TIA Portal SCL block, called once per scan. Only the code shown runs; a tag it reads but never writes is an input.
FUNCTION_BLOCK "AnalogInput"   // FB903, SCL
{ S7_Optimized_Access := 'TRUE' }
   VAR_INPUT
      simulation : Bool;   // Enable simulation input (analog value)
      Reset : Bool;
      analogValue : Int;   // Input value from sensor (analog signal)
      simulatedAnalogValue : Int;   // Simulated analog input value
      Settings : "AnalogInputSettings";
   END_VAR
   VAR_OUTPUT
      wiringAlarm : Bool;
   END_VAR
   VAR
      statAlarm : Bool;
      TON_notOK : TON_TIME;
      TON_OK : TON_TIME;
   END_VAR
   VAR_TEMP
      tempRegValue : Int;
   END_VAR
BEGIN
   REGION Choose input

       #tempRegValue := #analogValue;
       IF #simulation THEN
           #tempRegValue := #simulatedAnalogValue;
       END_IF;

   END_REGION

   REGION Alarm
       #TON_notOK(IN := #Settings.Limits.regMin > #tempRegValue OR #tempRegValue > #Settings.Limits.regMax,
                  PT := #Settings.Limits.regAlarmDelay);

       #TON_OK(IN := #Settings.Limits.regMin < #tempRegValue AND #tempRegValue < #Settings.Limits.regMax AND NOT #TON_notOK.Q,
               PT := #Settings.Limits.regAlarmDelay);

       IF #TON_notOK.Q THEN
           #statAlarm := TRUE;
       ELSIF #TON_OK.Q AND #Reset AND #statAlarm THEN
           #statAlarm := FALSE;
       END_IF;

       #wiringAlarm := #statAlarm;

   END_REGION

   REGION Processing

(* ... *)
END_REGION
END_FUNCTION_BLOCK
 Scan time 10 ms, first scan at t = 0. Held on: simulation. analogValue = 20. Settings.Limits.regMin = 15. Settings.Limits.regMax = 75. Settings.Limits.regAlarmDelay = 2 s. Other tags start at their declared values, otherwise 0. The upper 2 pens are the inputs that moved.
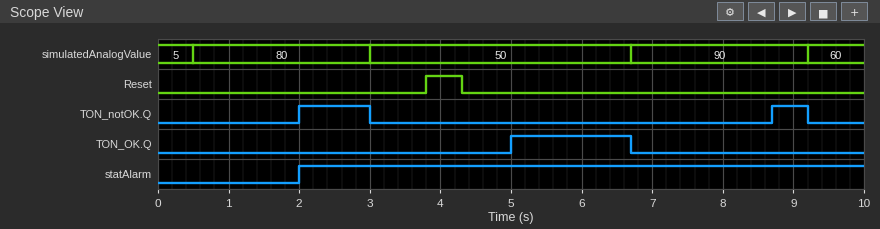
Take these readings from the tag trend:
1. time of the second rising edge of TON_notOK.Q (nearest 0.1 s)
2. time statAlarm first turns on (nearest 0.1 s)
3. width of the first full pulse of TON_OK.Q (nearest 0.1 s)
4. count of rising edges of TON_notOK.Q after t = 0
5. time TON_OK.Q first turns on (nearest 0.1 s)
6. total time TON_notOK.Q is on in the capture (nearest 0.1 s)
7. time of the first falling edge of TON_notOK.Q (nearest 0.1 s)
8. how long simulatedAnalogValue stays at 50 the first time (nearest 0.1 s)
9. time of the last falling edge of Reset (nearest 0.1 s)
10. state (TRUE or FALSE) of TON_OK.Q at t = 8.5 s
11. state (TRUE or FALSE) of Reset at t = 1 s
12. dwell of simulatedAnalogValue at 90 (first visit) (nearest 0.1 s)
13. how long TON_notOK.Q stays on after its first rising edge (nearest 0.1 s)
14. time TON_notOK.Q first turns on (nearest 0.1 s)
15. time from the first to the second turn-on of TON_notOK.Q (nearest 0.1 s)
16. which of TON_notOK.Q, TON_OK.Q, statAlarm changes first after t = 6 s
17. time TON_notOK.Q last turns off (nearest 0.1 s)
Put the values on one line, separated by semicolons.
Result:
8.7 s; 2.0 s; 1.7 s; 2; 5.0 s; 1.5 s; 3.0 s; 3.7 s; 4.3 s; FALSE; FALSE; 2.5 s; 1.0 s; 2.0 s; 6.7 s; TON_OK.Q; 9.2 s
